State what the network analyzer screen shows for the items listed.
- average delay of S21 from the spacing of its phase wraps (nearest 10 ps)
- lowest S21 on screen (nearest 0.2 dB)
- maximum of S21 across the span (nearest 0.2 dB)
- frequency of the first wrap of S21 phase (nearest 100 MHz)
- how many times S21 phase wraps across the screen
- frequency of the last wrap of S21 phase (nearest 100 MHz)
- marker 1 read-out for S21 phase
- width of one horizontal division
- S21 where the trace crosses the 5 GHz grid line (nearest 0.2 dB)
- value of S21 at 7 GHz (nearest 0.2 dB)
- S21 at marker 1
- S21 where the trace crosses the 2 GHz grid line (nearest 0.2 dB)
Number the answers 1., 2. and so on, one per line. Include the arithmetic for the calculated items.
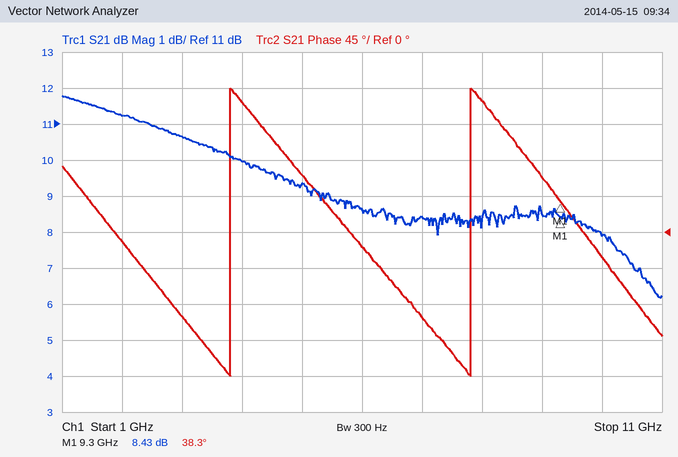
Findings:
1. 1 cycle / (7.8 GHz − 3.8 GHz) ≈ 250 ps
2. 6.2 dB
3. 11.8 dB
4. 3.8 GHz
5. 2
6. 7.8 GHz
7. 38.3°
8. 1 GHz
9. 9.4 dB
10. 8.4 dB
11. 8.43 dB
12. 11.2 dB
